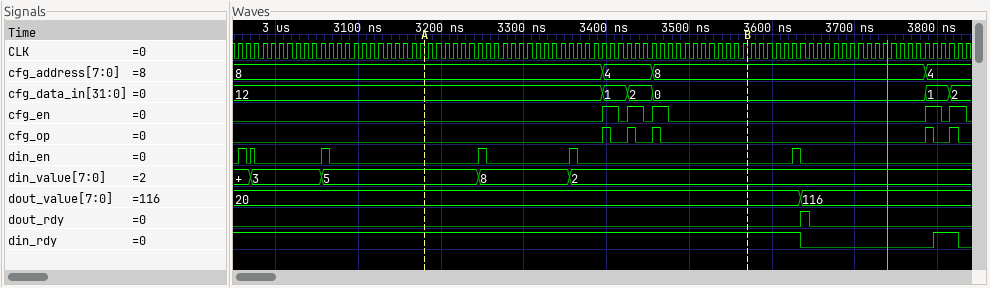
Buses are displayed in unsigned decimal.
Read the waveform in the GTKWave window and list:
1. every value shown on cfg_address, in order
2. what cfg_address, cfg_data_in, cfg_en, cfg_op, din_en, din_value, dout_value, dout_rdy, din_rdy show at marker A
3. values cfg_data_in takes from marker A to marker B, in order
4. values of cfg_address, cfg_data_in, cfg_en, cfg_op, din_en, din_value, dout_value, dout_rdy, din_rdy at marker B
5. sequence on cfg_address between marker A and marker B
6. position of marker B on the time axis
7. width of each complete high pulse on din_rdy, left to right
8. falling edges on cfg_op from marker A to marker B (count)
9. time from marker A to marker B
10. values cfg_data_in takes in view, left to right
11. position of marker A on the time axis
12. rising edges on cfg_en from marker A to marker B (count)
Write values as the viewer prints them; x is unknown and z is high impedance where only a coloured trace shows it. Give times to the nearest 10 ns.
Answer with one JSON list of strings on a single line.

["8, 4, 8, 4", "cfg_address=8, cfg_data_in=12, cfg_en=0, cfg_op=0, din_en=0, din_value=5, dout_value=20, dout_rdy=0, din_rdy=1", "12, 1, 2, 0", "cfg_address=8, cfg_data_in=0, cfg_en=0, cfg_op=0, din_en=0, din_value=2, dout_value=20, dout_rdy=0, din_rdy=1", "8, 4, 8", "3570 ns", "30 ns", "3", "390 ns", "12, 1, 2, 0, 1, 2", "3180 ns", "3"]
